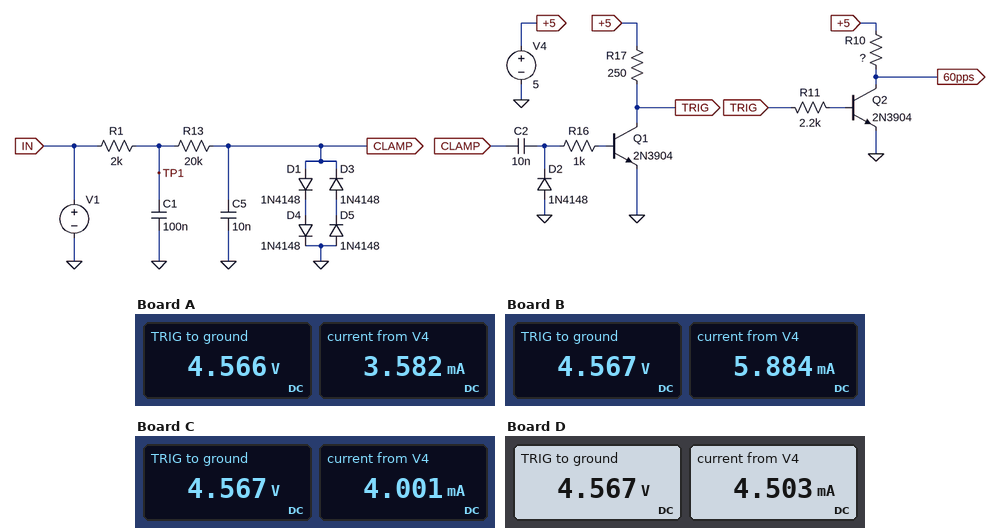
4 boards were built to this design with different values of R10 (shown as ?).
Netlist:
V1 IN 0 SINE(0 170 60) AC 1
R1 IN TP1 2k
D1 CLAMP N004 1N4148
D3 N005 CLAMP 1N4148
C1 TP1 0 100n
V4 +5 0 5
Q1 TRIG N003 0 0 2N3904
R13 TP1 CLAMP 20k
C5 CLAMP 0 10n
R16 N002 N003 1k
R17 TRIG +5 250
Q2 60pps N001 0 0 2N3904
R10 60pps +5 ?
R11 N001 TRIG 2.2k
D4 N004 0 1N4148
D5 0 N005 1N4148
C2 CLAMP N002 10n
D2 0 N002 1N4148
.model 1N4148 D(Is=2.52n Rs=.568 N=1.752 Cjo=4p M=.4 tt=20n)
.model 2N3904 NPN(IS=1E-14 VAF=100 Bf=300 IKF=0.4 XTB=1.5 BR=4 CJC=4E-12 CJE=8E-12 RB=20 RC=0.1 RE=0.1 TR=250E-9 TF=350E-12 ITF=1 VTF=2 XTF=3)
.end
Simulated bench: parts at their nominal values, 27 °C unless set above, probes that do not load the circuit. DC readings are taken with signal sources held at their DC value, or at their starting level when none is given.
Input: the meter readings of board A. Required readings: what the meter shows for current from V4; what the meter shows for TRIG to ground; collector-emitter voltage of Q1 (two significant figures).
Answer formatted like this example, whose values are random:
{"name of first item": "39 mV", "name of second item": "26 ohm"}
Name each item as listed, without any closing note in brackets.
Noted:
{"what the meter shows for current from V4": "3.582 mA", "what the meter shows for TRIG to ground": "4.566 V", "collector-emitter voltage of Q1": "4.6 V"}
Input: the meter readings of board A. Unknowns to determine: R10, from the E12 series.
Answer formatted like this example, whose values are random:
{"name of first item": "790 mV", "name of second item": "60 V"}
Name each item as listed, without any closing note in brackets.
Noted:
{"R10, from the E12 series": "2.7 kΩ"}
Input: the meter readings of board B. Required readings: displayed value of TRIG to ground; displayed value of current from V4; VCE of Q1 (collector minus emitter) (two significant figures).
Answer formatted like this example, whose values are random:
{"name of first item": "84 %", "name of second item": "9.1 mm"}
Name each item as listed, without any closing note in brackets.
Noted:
{"displayed value of TRIG to ground": "4.567 V", "displayed value of current from V4": "5.884 mA", "VCE of Q1 (collector minus emitter)": "4.6 V"}
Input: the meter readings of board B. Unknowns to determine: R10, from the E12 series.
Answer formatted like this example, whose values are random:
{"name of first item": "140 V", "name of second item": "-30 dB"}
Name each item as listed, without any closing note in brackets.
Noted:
{"R10, from the E12 series": "1.2 kΩ"}
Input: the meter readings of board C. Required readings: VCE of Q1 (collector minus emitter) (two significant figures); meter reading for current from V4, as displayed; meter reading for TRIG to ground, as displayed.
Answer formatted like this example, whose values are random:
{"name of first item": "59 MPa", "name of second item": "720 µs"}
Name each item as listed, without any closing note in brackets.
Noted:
{"VCE of Q1 (collector minus emitter)": "4.6 V", "meter reading for current from V4, as displayed": "4.001 mA", "meter reading for TRIG to ground, as displayed": "4.567 V"}
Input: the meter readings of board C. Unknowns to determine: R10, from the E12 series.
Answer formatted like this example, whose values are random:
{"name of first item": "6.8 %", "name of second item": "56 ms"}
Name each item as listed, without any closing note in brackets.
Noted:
{"R10, from the E12 series": "2.2 kΩ"}
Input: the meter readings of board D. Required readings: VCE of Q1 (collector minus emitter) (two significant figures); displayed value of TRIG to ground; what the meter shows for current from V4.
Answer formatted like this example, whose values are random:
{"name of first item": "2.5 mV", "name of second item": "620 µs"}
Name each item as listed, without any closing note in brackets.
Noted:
{"VCE of Q1 (collector minus emitter)": "4.6 V", "displayed value of TRIG to ground": "4.567 V", "what the meter shows for current from V4": "4.503 mA"}
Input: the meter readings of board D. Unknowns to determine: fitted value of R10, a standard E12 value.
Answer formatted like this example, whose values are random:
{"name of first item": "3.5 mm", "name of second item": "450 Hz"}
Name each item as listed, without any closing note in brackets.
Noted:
{"fitted value of R10, a standard E12 value": "1.8 kΩ"}
